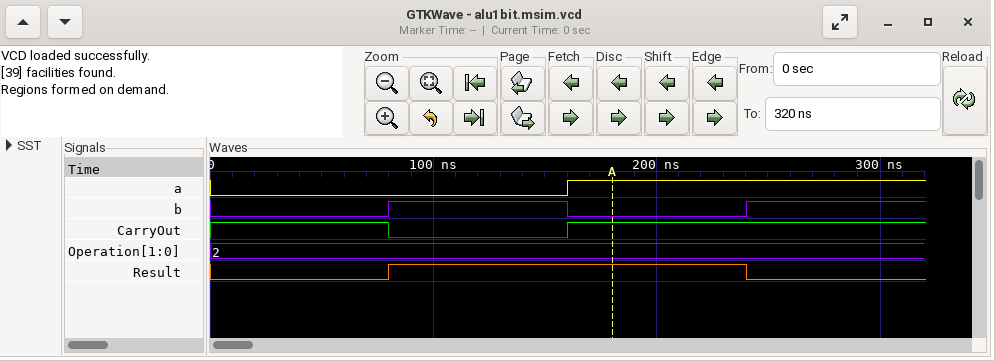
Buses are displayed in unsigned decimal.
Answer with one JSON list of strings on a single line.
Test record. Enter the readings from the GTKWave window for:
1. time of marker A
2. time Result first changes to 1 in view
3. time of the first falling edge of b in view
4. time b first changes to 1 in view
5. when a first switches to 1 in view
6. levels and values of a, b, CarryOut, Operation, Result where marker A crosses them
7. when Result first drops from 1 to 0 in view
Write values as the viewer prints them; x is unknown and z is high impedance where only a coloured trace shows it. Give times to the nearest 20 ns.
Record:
["180 ns", "80 ns", "160 ns", "80 ns", "160 ns", "a=1, b=0, CarryOut=1, Operation=2, Result=1", "240 ns"]
